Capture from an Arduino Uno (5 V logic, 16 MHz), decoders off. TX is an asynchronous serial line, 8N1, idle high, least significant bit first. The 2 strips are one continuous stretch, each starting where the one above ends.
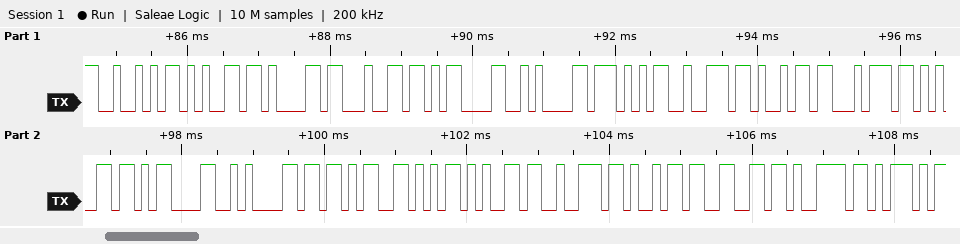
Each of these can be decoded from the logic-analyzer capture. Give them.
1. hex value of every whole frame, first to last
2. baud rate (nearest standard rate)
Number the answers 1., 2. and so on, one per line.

1. 52 65 61 64 0D 0A 57 72 69 74 65 0D 0A 5B 56 65 72 69 66 79 5D
2. 9600 baud
